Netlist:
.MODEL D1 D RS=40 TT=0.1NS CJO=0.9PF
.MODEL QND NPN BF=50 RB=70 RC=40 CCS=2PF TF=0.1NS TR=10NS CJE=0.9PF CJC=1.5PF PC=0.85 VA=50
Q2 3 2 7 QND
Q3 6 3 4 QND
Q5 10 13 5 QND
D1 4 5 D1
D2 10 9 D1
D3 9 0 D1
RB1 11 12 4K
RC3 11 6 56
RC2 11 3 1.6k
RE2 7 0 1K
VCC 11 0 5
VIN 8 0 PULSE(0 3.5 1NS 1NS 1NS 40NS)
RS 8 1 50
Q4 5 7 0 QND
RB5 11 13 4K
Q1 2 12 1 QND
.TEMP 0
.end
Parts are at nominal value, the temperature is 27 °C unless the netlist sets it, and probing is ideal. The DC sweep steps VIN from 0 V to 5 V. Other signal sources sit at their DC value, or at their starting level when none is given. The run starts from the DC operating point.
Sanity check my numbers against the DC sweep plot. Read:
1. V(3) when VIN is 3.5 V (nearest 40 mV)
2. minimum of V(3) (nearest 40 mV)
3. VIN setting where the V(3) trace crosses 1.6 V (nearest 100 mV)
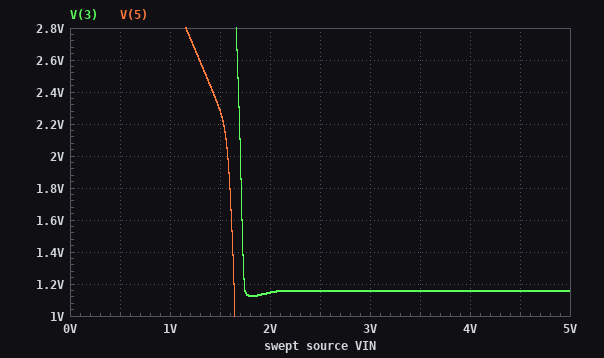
1.16 V
1.12 V
1.7 V
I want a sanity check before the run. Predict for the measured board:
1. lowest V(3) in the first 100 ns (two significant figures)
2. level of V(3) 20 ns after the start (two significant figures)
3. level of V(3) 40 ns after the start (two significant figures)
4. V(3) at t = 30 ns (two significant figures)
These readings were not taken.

130 mV
1.2 V
1.2 V
1.2 V
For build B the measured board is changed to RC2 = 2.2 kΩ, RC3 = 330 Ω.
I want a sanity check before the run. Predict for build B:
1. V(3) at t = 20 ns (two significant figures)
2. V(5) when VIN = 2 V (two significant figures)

1.1 V
63 mV
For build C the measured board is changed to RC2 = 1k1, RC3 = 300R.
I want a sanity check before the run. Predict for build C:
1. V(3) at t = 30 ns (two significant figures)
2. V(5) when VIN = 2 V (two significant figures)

1.3 V
61 mV
